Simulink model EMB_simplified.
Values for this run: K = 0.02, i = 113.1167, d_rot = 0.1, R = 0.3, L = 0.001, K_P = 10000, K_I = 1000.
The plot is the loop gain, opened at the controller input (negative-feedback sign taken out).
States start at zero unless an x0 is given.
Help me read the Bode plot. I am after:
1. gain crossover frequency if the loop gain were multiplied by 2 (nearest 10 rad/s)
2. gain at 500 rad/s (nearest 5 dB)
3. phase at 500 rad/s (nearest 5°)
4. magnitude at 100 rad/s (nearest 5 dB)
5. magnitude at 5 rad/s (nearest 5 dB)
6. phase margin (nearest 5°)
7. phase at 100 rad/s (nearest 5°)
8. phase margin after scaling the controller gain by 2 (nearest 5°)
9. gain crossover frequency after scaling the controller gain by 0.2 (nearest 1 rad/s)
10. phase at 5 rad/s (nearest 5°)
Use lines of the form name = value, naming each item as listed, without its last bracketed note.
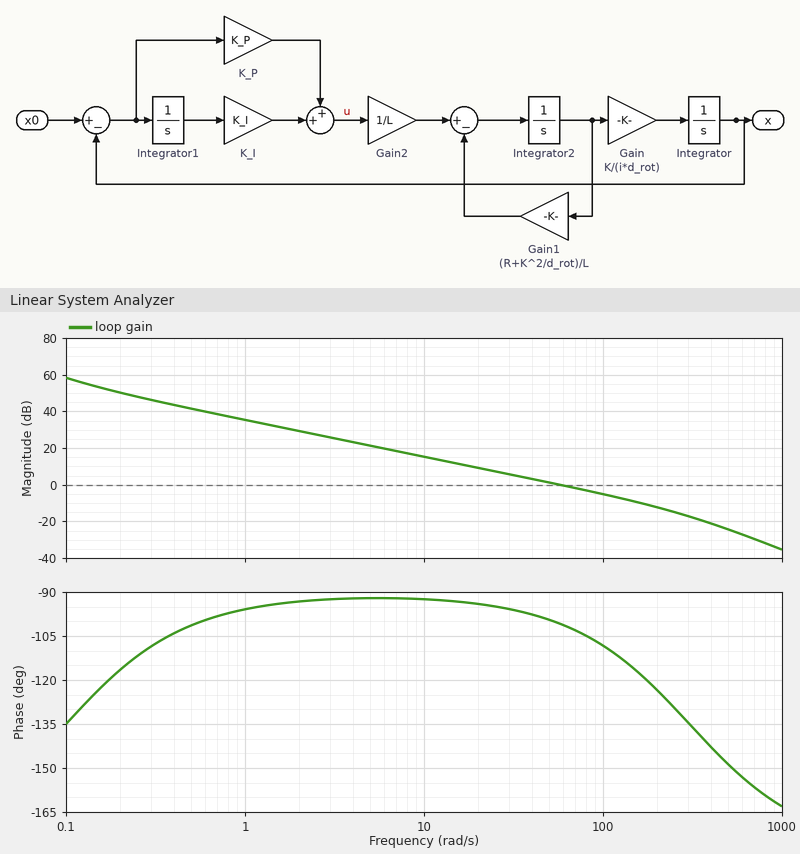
gain crossover frequency if the loop gain were multiplied by 2 = 110 rad/s
gain at 500 rad/s = -25 dB
phase at 500 rad/s = -150°
magnitude at 100 rad/s = -5 dB
magnitude at 5 rad/s = 20 dB
phase margin = 80°
phase at 100 rad/s = -110°
phase margin after scaling the controller gain by 2 = 70°
gain crossover frequency after scaling the controller gain by 0.2 = 12 rad/s
phase at 5 rad/s = -90°
